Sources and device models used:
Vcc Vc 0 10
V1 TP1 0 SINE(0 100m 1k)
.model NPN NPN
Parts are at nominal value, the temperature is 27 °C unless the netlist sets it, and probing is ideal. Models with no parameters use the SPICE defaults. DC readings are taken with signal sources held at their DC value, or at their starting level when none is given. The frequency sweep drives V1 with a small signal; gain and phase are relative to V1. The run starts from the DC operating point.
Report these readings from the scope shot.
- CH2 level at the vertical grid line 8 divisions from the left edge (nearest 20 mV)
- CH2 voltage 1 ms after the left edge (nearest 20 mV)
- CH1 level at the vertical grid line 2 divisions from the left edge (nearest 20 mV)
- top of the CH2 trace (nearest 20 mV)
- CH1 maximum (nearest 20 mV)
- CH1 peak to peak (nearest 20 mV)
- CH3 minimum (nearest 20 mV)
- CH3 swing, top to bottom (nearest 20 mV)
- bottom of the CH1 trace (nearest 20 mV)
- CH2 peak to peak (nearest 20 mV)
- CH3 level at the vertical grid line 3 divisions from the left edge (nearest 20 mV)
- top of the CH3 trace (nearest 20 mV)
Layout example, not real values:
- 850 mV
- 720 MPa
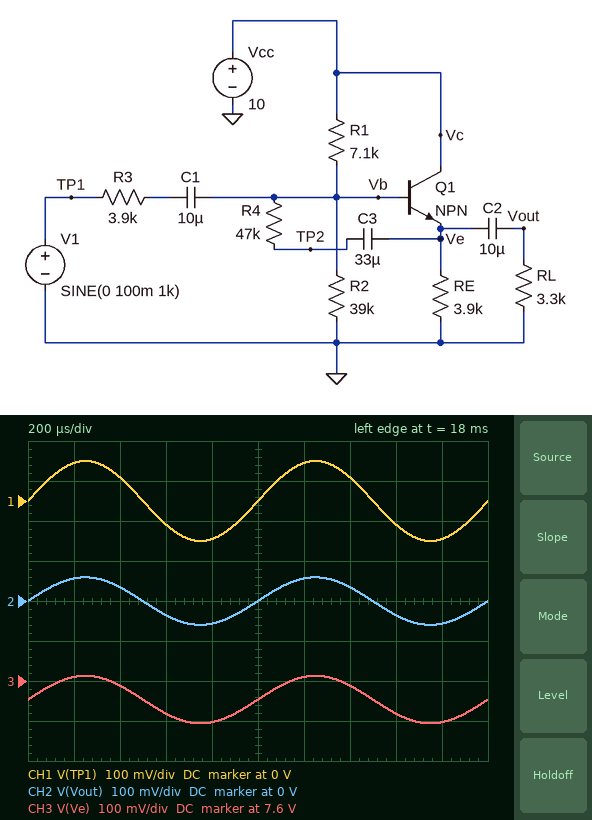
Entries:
- -40 mV
- 0 V
- 60 mV
- 60 mV
- 100 mV
- 200 mV
- 7.50 V
- 120 mV
- -100 mV
- 120 mV
- 7.52 V
- 7.62 V
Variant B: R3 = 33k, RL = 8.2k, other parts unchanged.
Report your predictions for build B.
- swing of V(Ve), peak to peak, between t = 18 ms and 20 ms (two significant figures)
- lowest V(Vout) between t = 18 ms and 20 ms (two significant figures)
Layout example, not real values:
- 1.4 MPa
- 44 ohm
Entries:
- 30 mV
- -15 mV
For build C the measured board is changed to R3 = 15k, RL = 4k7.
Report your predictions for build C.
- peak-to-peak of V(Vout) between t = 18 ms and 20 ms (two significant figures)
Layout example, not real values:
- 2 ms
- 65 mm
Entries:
- 56 mV
